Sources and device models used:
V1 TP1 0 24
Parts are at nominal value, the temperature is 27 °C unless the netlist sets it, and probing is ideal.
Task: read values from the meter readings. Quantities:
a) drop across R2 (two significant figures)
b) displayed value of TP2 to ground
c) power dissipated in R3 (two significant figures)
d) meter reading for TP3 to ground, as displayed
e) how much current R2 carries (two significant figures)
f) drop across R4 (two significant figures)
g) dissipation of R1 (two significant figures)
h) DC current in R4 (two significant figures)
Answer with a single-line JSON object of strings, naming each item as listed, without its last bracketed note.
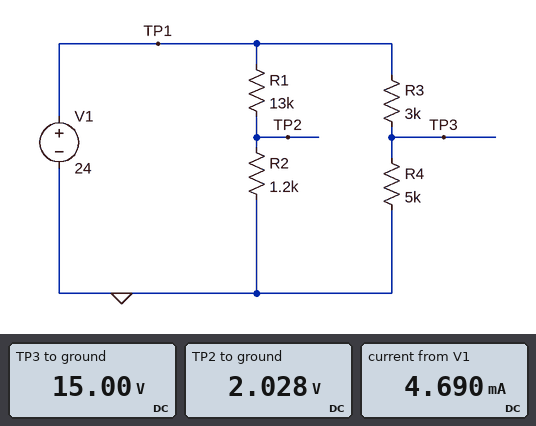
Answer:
{"drop across R2": "2.0 V", "displayed value of TP2 to ground": "2.028 V", "power dissipated in R3": "27 mW", "meter reading for TP3 to ground, as displayed": "15.00 V", "how much current R2 carries": "1.7 mA", "drop across R4": "15 V", "dissipation of R1": "37 mW", "DC current in R4": "3.0 mA"}
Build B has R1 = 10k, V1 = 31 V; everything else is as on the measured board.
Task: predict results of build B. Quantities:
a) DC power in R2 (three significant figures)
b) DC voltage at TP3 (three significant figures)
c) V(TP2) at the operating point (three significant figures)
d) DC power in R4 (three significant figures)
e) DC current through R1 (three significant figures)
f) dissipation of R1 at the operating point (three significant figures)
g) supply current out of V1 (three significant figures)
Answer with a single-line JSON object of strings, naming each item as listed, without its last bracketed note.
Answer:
{"DC power in R2": "9.19 mW", "DC voltage at TP3": "19.4 V", "V(TP2) at the operating point": "3.32 V", "DC power in R4": "75.1 mW", "DC current through R1": "2.77 mA", "dissipation of R1 at the operating point": "76.6 mW", "supply current out of V1": "6.64 mA"}
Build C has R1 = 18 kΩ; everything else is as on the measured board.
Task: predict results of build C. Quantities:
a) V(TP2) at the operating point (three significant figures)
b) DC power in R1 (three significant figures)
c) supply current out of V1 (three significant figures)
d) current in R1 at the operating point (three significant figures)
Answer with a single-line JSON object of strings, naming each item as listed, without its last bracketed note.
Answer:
{"V(TP2) at the operating point": "1.50 V", "DC power in R1": "28.1 mW", "supply current out of V1": "4.25 mA", "current in R1 at the operating point": "1.25 mA"}
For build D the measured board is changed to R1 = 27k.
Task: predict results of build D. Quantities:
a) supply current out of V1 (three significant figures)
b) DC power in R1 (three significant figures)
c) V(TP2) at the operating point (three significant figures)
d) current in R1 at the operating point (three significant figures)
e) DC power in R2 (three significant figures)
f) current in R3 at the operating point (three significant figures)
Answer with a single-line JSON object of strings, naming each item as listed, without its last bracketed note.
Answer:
{"supply current out of V1": "3.85 mA", "DC power in R1": "19.6 mW", "V(TP2) at the operating point": "1.02 V", "current in R1 at the operating point": "851 µA", "DC power in R2": "869 µW", "current in R3 at the operating point": "3.00 mA"}
